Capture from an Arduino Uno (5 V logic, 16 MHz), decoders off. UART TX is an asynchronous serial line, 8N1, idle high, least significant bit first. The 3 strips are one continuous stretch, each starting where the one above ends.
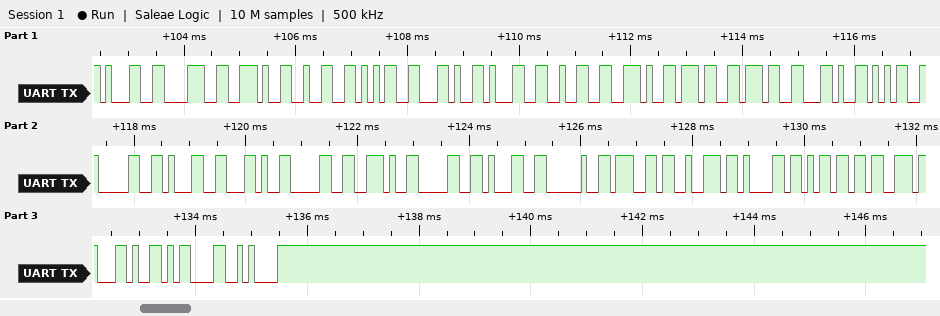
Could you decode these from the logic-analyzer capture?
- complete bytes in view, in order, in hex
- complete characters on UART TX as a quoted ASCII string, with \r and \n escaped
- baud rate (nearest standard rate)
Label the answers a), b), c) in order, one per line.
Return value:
a) 31 38 2E 32 35 2C 31 32 2E 37 37 2C 35 30 31 2C 30 2E 30 31 20 67 72 61 6D 73 2C 0D 0A
b) "18.25,12.77,501,0.01 grams,\r\n"
c) 9600 baud
